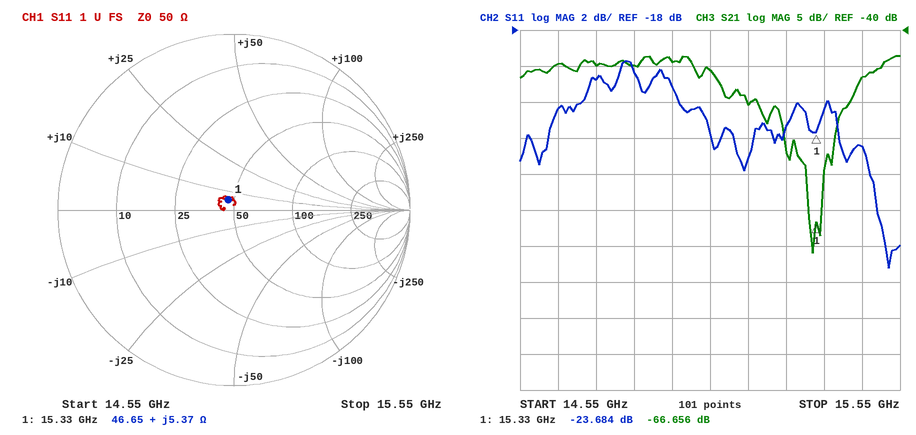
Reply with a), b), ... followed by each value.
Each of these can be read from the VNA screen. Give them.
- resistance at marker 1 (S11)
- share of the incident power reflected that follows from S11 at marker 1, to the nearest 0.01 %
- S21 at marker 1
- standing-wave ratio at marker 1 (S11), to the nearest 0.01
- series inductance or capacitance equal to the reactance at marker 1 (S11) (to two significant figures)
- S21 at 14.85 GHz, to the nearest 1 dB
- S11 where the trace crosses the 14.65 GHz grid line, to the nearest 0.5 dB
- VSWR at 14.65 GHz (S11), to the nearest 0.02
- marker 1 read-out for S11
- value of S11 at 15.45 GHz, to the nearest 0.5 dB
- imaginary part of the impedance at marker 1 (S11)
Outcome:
a) 46.65 Ω
b) 0.43 %
c) -66.656 dB
d) 1.14
e) 56 pH
f) -45 dB
g) -22.5 dB
h) 1.16
i) -23.684 dB
j) -24.5 dB
k) +5.37 Ω
